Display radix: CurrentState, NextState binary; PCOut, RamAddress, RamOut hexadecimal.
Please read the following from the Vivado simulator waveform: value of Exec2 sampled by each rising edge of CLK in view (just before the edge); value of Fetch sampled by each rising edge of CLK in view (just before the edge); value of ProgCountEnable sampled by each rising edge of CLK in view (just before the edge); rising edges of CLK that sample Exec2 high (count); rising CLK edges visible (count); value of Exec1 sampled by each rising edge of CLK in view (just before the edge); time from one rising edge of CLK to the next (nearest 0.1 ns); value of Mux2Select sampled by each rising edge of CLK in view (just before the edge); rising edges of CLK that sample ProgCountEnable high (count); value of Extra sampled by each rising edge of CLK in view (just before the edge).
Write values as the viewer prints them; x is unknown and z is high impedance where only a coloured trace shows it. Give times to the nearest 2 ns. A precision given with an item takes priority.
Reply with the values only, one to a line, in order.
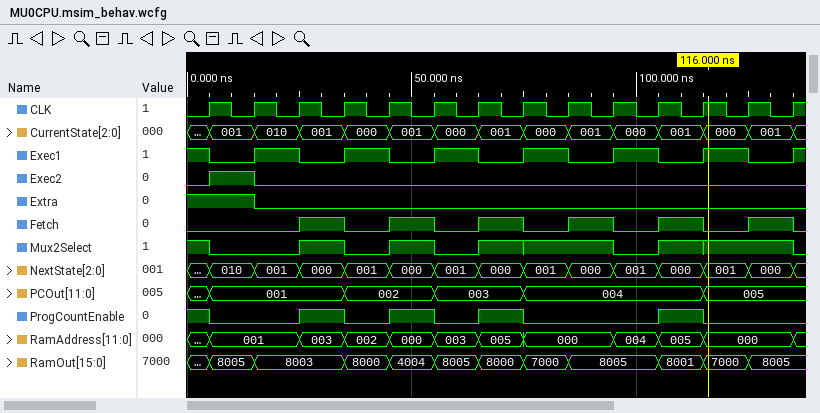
0 1 0 0 0 0 0 0 0 0 0 0 0 0
0 0 0 1 0 1 0 1 0 1 0 1 0 1
1 0 0 1 0 1 0 1 0 0 0 1 0 0
1
14
1 0 1 0 1 0 1 0 1 0 1 0 1 0
10 ns
1 0 0 1 0 1 0 1 1 1 0 1 1 1
5
1 1 0 0 0 0 0 0 0 0 0 0 0 0
